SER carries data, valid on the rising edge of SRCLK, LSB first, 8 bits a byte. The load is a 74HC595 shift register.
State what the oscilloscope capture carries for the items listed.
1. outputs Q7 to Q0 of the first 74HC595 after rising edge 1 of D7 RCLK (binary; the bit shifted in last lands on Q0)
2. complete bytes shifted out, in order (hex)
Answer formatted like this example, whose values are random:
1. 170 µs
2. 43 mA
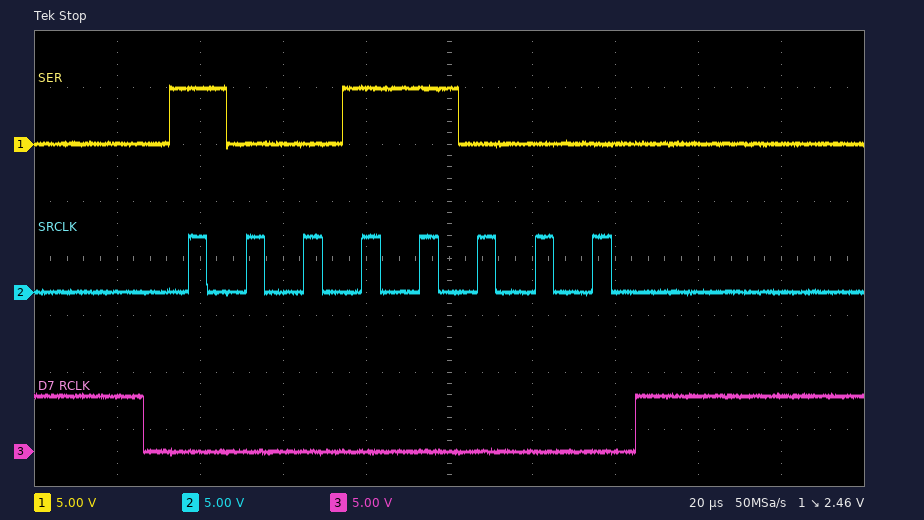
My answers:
1. 10011000
2. 0x19
